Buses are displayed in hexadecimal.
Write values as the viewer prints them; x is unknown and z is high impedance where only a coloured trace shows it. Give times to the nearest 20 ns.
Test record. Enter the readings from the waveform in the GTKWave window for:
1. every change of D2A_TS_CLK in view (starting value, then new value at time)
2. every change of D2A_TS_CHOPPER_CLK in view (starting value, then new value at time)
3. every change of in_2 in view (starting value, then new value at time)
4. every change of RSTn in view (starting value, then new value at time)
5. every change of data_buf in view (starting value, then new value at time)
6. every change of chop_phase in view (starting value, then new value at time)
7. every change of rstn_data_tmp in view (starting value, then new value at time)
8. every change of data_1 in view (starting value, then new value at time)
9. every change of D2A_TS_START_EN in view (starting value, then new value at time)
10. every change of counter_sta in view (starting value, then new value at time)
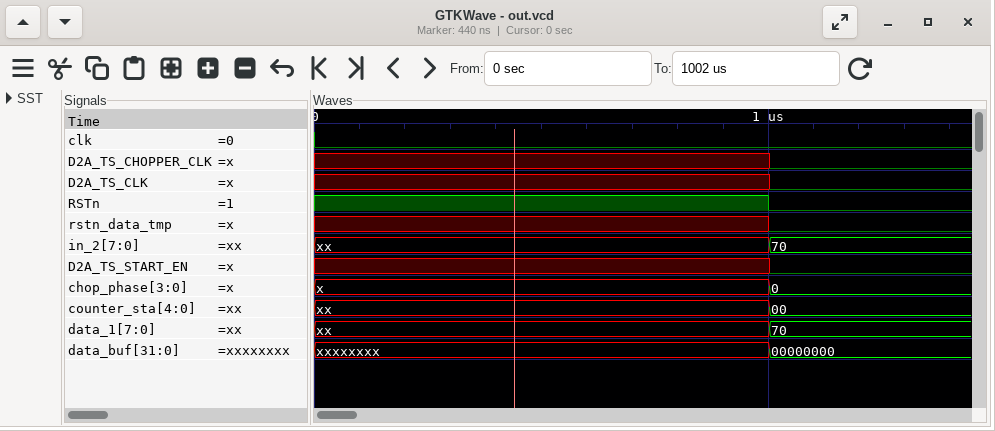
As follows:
x, 0 at 1000 ns
x, 0 at 1000 ns
xx, 70 at 1000 ns
1, 0 at 1000 ns
xxxxxxxx, 00000000 at 1000 ns
x, 0 at 1000 ns
x, 0 at 1000 ns
xx, 70 at 1000 ns
x, 0 at 1000 ns
xx, 00 at 1000 ns
